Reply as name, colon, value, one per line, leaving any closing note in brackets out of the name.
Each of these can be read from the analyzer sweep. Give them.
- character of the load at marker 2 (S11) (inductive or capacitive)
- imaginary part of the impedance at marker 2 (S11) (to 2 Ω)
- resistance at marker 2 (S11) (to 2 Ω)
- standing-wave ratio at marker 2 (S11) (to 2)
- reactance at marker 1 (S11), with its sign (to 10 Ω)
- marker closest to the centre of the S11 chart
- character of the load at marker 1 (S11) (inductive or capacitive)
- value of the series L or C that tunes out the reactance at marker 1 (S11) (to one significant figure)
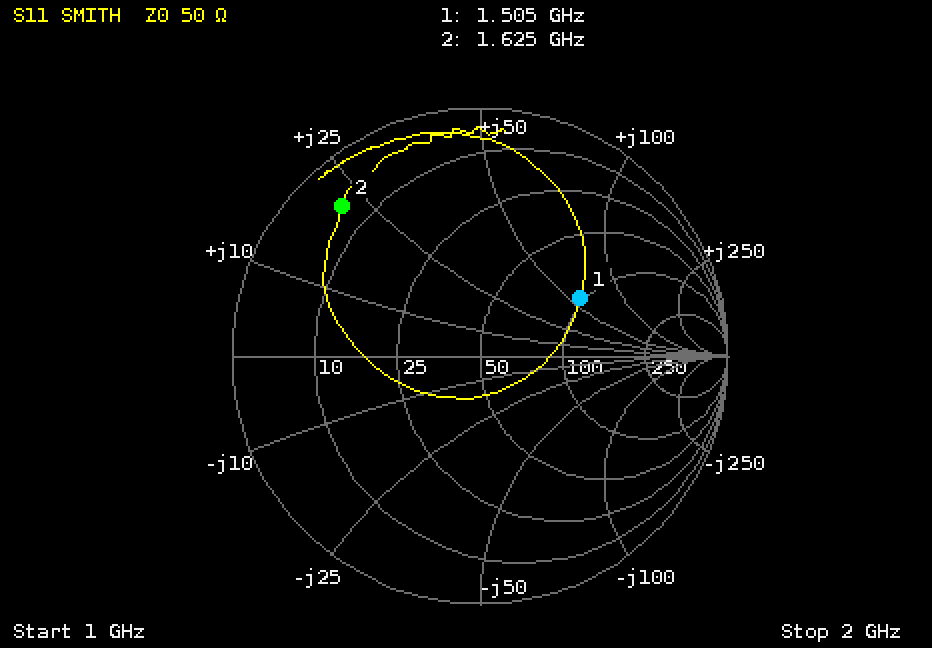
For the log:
character of the load at marker 2 (S11): inductive
imaginary part of the impedance at marker 2 (S11): +22 Ω
resistance at marker 2 (S11): 6 Ω
standing-wave ratio at marker 2 (S11): 10
reactance at marker 1 (S11), with its sign: +60 Ω
marker closest to the centre of the S11 chart: marker 1
character of the load at marker 1 (S11): inductive
value of the series L or C that tunes out the reactance at marker 1 (S11): 2 pF
